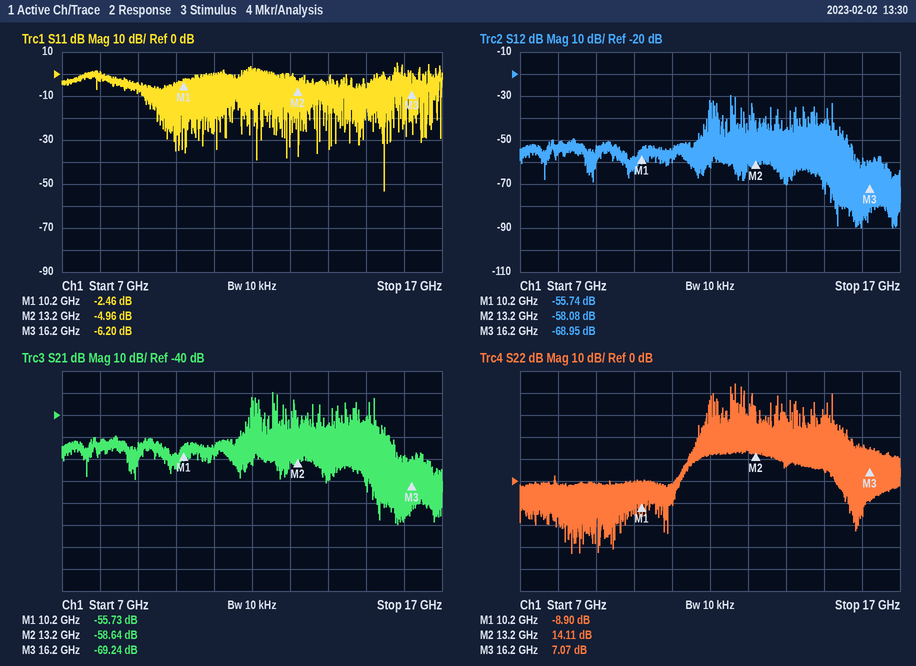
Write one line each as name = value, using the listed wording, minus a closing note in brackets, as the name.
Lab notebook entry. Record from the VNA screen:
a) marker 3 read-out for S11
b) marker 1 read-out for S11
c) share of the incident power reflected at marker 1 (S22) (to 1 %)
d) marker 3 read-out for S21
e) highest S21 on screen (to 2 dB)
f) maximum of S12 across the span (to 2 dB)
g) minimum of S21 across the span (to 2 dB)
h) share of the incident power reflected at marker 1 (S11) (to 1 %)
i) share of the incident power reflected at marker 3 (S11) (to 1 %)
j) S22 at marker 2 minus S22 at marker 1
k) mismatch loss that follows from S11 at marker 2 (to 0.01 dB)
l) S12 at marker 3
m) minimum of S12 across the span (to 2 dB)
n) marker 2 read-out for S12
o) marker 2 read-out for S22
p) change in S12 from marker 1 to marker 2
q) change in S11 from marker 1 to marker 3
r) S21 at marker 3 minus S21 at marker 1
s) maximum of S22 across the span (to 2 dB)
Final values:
marker 3 read-out for S11 = -6.20 dB
marker 1 read-out for S11 = -2.46 dB
share of the incident power reflected at marker 1 (S22) = 13 %
marker 3 read-out for S21 = -69.24 dB
highest S21 on screen = -30 dB
maximum of S12 across the span = -30 dB
minimum of S21 across the span = -90 dB
share of the incident power reflected at marker 1 (S11) = 57 %
share of the incident power reflected at marker 3 (S11) = 24 %
S22 at marker 2 minus S22 at marker 1 = 23.01 dB
mismatch loss that follows from S11 at marker 2 = 1.67 dB
S12 at marker 3 = -68.95 dB
minimum of S12 across the span = -90 dB
marker 2 read-out for S12 = -58.08 dB
marker 2 read-out for S22 = 14.11 dB
change in S12 from marker 1 to marker 2 = -2.34 dB
change in S11 from marker 1 to marker 3 = -3.74 dB
S21 at marker 3 minus S21 at marker 1 = -13.51 dB
maximum of S22 across the span = 44 dB
